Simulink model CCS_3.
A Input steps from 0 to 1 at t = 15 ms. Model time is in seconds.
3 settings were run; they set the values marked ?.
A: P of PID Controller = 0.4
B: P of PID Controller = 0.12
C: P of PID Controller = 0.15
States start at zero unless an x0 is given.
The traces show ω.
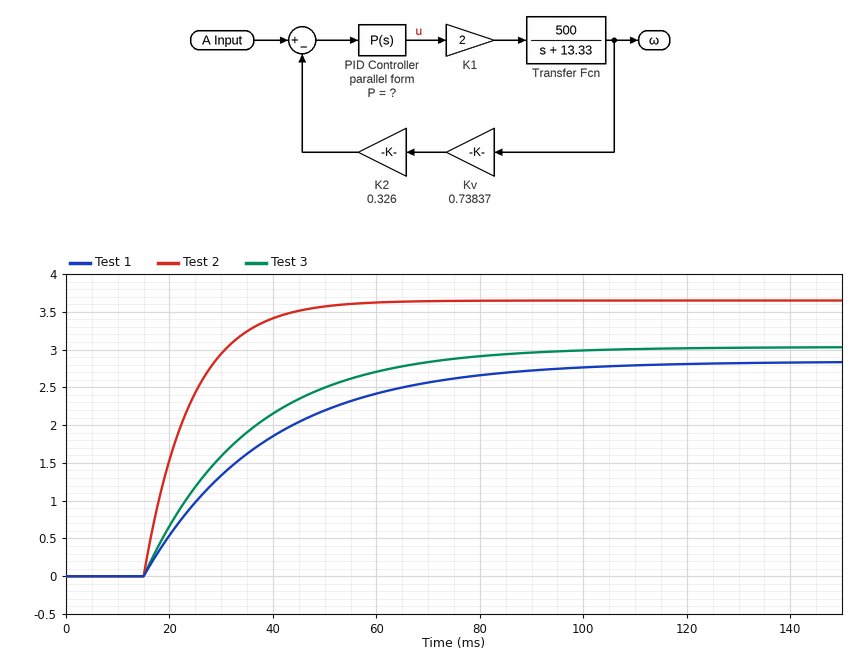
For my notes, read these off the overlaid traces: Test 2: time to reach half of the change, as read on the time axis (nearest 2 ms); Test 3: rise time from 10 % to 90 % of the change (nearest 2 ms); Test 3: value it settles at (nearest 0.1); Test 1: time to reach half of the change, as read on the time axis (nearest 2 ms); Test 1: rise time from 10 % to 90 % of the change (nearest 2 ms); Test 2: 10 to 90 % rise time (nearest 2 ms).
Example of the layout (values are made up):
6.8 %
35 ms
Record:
22 ms
44 ms
3.0
32 ms
52 ms
20 ms
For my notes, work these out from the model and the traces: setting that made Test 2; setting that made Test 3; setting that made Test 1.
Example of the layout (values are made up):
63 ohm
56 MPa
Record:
A
C
B
